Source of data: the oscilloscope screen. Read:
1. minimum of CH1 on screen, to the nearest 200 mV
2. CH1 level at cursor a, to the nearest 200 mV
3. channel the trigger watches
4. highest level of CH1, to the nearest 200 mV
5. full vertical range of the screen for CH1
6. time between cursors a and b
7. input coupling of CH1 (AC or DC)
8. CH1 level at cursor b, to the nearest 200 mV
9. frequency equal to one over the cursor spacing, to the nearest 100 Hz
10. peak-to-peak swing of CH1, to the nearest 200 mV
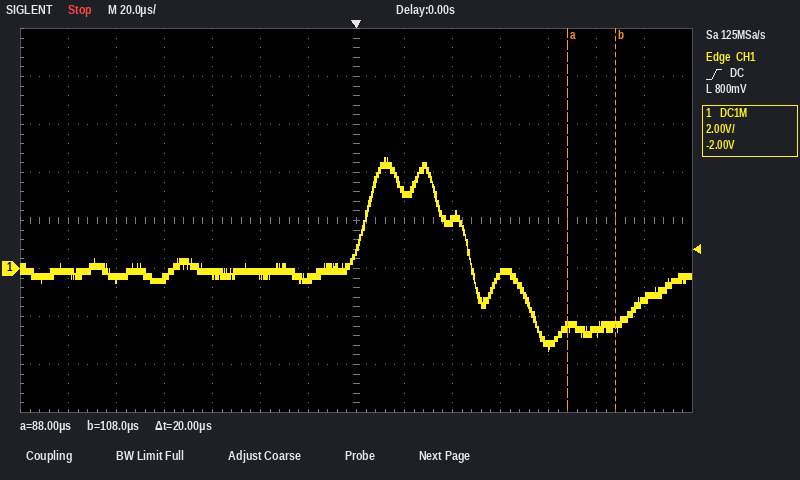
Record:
-3.4 V
-2.4 V
CH1
4.6 V
16 V
20 µs
DC
-2.4 V
50.0 kHz
8.0 V
